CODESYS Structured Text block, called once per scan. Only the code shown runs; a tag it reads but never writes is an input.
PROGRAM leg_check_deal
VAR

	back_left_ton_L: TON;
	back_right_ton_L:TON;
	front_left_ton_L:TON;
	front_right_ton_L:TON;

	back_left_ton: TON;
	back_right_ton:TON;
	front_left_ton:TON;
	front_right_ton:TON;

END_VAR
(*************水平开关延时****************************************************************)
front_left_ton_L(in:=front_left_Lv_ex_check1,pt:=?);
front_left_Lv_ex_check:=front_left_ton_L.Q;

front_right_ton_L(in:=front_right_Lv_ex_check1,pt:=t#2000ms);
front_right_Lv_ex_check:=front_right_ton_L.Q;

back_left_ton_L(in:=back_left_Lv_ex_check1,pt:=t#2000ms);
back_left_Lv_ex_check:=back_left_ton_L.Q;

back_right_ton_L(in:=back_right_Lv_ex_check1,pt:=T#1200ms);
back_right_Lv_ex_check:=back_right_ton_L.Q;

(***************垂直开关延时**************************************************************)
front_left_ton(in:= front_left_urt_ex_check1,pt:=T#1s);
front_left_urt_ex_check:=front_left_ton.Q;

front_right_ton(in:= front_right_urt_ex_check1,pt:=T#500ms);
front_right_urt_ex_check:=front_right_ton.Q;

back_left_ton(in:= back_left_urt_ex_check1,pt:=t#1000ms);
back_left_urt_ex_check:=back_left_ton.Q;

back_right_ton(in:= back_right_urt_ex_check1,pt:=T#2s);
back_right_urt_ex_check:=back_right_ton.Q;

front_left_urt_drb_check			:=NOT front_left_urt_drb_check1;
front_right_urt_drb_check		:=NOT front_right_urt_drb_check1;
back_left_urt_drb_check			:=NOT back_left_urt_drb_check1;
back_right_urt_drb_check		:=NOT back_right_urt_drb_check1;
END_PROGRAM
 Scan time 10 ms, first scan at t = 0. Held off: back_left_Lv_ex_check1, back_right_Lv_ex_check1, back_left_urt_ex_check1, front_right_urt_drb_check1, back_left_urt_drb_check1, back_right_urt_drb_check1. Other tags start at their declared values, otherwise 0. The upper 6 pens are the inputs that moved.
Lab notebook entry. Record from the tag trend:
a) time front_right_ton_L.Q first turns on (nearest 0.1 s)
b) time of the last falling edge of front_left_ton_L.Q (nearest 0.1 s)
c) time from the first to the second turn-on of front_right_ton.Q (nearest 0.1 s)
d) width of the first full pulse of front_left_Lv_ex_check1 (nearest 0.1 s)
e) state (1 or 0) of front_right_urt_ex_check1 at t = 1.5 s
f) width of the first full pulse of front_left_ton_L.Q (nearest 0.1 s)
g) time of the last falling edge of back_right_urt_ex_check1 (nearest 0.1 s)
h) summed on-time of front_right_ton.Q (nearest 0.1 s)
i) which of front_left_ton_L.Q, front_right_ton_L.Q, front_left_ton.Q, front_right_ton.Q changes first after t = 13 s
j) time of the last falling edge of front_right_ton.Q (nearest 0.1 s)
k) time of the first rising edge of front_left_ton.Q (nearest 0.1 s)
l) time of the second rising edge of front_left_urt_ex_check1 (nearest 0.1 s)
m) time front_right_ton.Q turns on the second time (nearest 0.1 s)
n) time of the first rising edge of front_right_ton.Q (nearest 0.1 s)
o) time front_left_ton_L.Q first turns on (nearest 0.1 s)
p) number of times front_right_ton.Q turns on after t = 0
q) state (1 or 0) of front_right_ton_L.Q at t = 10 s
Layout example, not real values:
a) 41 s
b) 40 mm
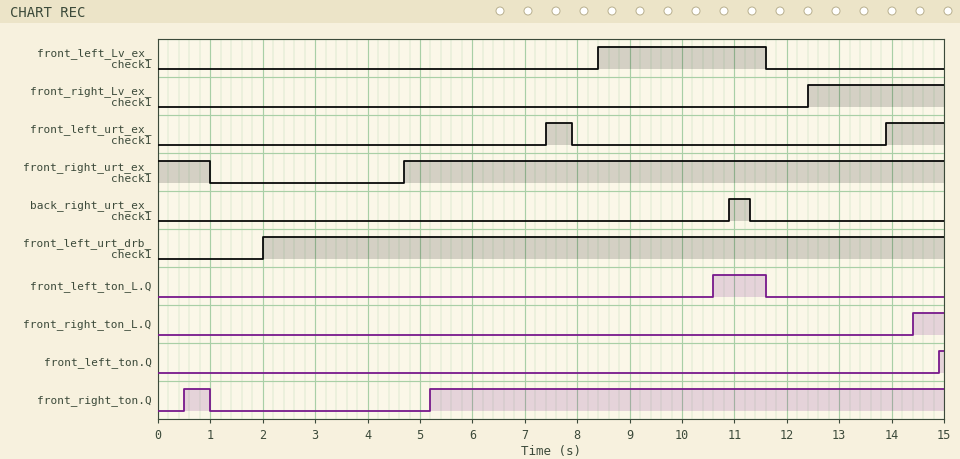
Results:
a) 14.4 s
b) 11.6 s
c) 4.7 s
d) 3.2 s
e) 0
f) 1.0 s
g) 11.3 s
h) 10.3 s
i) front_right_ton_L.Q
j) 1.0 s
k) 14.9 s
l) 13.9 s
m) 5.2 s
n) 0.5 s
o) 10.6 s
p) 2
q) 0
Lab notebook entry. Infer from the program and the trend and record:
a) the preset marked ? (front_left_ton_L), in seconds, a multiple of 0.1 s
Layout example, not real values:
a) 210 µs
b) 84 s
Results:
a) 2.2 s
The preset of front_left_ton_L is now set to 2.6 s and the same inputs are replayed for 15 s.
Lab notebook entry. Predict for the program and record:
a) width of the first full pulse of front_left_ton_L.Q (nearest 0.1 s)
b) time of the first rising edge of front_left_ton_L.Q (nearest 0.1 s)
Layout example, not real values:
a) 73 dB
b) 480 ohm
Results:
a) 0.6 s
b) 11.0 s
